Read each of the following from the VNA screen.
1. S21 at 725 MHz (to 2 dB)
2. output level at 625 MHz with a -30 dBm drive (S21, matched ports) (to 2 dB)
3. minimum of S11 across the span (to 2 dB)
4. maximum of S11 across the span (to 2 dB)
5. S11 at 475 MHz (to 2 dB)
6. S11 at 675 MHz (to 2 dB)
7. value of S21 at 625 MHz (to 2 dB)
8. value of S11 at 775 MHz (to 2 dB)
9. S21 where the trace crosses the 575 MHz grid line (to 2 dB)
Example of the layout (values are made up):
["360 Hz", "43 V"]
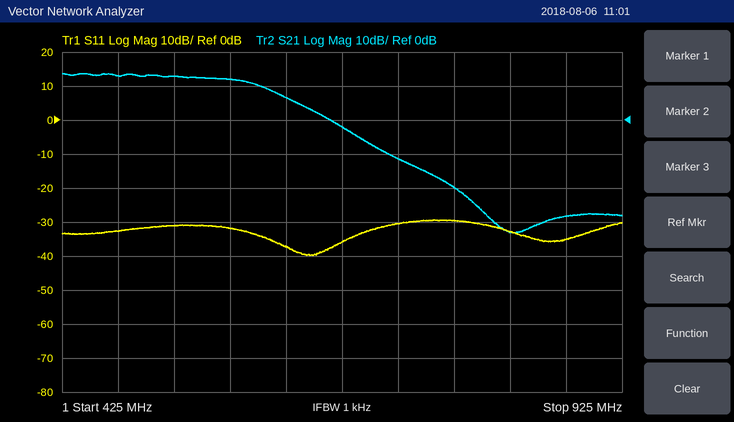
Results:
["-12 dB", "-24 dBm", "-40 dB", "-30 dB", "-32 dB", "-36 dB", "6 dB", "-30 dB", "12 dB"]
